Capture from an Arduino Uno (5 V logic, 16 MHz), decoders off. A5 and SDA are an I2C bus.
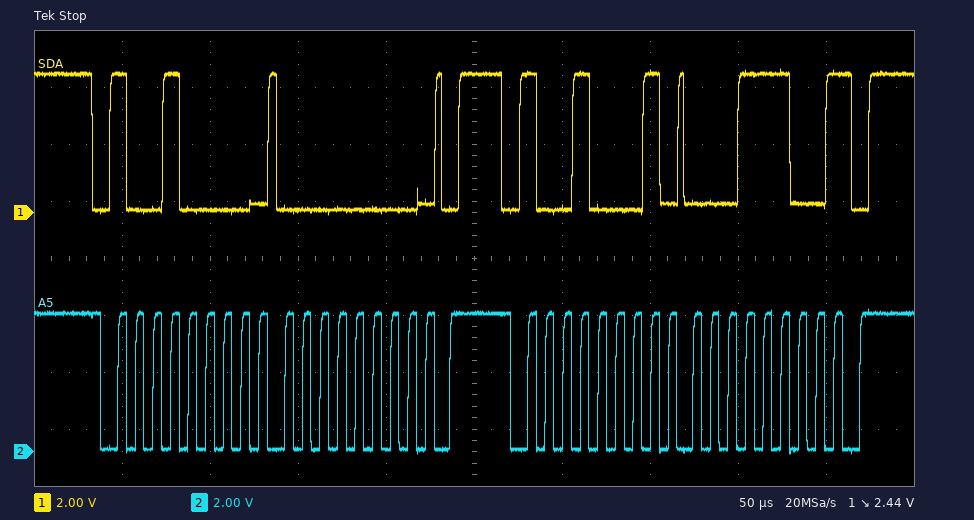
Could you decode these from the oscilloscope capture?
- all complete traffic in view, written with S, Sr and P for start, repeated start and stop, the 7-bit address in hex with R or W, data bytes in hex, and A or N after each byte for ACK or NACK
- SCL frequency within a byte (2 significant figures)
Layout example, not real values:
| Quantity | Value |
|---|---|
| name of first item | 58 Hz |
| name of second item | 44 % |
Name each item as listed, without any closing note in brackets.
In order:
| Quantity | Value |
|---|---|
| all complete traffic in view, written with S, Sr and P for start, repeated start and stop, the 7-bit address in hex with R or W, data bytes in hex, and A or N after each byte for ACK or NACK | S 48W A 00 A P S 48R A 1C N P |
| SCL frequency within a byte | 100 kHz |
